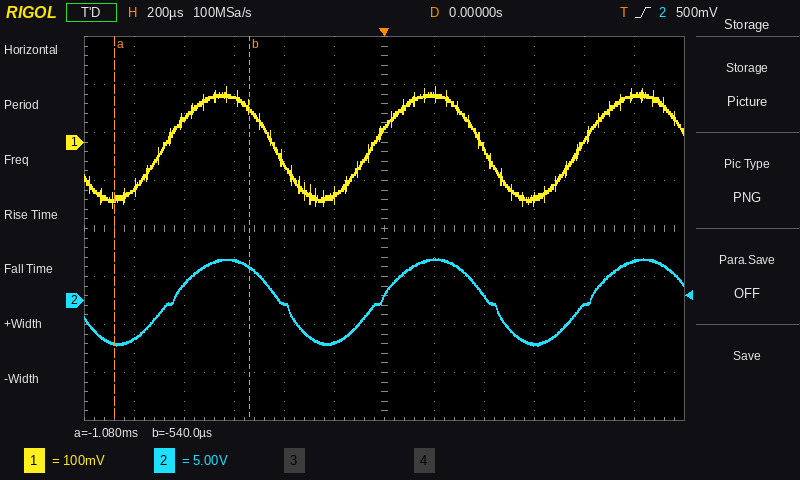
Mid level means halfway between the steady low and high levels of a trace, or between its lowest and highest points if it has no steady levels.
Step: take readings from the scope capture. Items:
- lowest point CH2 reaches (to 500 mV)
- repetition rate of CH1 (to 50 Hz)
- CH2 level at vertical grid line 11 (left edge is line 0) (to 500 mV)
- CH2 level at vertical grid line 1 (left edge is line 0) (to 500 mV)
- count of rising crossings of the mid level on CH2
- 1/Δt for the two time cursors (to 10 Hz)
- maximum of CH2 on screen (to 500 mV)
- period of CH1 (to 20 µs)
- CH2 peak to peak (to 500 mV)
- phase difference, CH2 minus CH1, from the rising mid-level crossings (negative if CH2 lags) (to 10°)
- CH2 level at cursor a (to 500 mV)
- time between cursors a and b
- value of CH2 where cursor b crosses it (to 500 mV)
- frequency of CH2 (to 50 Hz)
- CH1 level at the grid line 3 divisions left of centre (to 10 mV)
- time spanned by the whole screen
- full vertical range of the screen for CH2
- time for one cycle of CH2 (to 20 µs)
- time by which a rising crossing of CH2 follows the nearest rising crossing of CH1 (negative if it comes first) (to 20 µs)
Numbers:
-4.5 V
1.20 kHz
4.0 V
-4.0 V
3
1.85 kHz
4.5 V
840 µs
9.0 V
-20°
-4.5 V
540 µs
3.5 V
1.20 kHz
90 mV
2.4 ms
40 V
840 µs
+40 µs
